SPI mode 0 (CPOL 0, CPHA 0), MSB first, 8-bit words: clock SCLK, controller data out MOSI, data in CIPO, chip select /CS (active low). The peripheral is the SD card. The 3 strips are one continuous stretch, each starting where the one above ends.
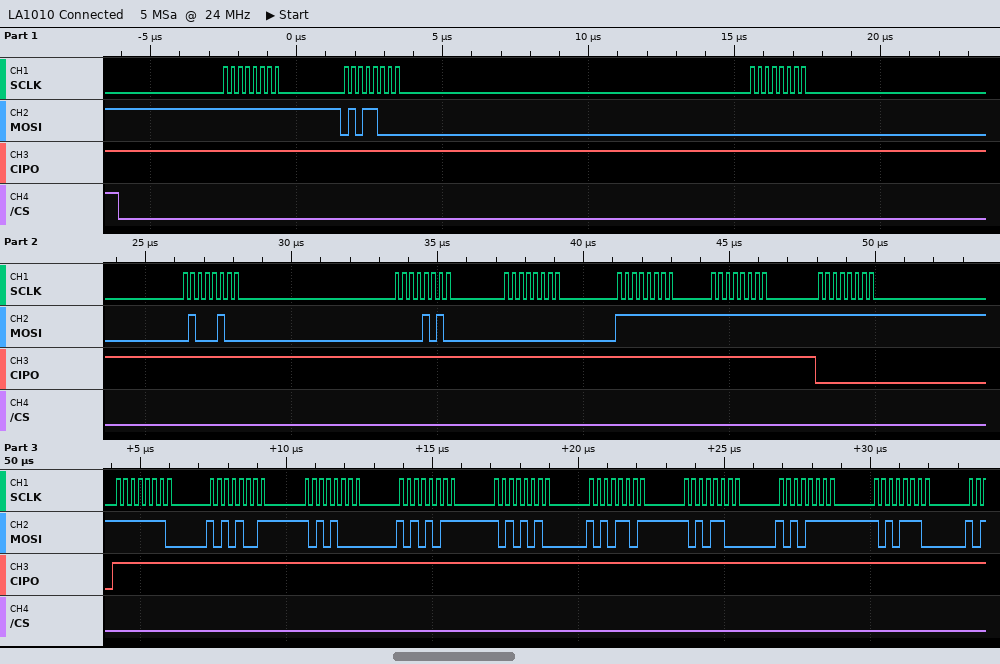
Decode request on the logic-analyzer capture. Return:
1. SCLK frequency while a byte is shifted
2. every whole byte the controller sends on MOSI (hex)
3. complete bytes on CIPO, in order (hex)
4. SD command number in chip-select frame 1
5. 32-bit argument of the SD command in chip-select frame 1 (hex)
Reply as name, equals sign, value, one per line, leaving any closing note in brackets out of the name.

SCLK frequency while a byte is shifted = 4 MHz
every whole byte the controller sends on MOSI = 0xFF 0x58 0x00 0x44 0x0A 0x00 0xFF 0xFF 0xFF 0xFE 0xA9 0xA8 0xAB 0xAA 0xAD 0xAC 0xAF 0xAE
complete bytes on CIPO, in order = 0xFF 0xFF 0xFF 0xFF 0xFF 0xFF 0xFF 0xFF 0x00 0xFF 0xFF 0xFF 0xFF 0xFF 0xFF 0xFF 0xFF 0xFF
SD command number in chip-select frame 1 = CMD24
32-bit argument of the SD command in chip-select frame 1 = 0x00440A00
